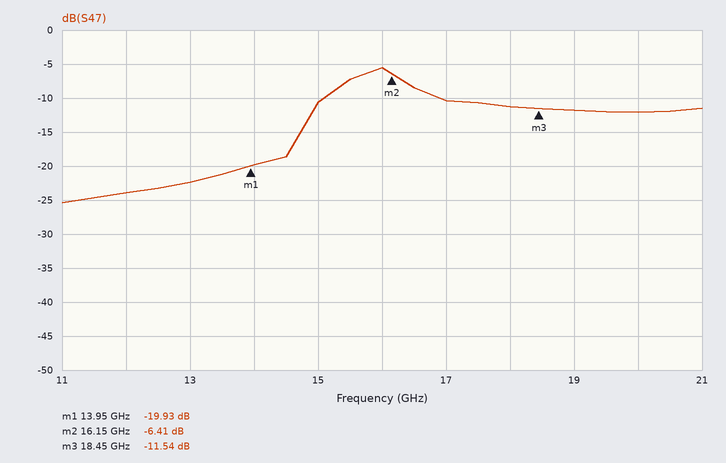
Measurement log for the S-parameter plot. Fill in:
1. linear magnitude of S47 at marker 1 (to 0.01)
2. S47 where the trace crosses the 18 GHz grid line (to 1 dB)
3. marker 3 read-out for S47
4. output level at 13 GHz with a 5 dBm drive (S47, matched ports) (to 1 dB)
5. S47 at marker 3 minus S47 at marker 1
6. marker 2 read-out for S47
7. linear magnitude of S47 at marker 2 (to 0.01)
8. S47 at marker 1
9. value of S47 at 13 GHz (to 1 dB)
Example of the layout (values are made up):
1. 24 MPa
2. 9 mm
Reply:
1. 0.10
2. -11 dB
3. -11.54 dB
4. -17 dBm
5. 8.39 dB
6. -6.41 dB
7. 0.48
8. -19.93 dB
9. -22 dB
